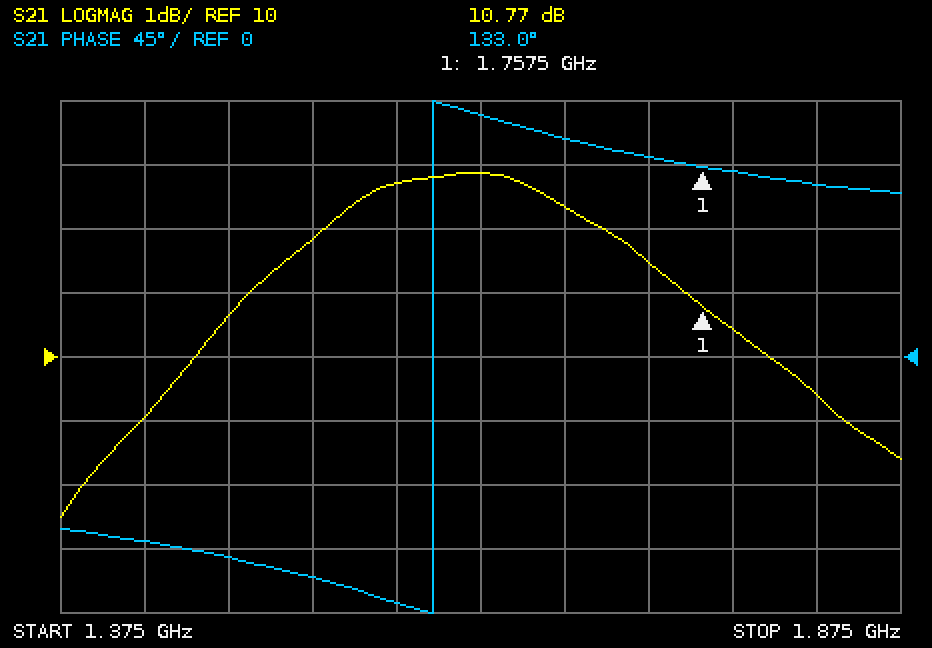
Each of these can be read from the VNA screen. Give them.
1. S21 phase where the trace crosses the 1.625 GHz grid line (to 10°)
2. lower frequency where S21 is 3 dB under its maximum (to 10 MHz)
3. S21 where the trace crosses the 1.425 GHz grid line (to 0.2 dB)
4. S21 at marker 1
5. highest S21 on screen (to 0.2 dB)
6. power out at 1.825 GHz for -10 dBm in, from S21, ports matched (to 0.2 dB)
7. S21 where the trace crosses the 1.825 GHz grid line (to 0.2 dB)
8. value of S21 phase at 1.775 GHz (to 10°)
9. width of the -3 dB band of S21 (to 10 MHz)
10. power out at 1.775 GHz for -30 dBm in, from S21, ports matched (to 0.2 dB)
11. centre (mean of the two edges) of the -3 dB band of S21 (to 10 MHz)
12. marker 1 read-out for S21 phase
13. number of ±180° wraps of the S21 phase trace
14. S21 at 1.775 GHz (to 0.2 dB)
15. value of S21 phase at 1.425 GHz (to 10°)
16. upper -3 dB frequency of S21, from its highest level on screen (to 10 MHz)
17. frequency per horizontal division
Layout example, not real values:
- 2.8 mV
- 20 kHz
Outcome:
- 170°
- 1.45 GHz
- 9.0 dB
- 10.77 dB
- 12.8 dB
- -0.6 dBm
- 9.4 dB
- 130°
- 350 MHz
- -19.6 dBm
- 1.63 GHz
- 133.0°
- 1
- 10.4 dB
- -130°
- 1.80 GHz
- 50 MHz
